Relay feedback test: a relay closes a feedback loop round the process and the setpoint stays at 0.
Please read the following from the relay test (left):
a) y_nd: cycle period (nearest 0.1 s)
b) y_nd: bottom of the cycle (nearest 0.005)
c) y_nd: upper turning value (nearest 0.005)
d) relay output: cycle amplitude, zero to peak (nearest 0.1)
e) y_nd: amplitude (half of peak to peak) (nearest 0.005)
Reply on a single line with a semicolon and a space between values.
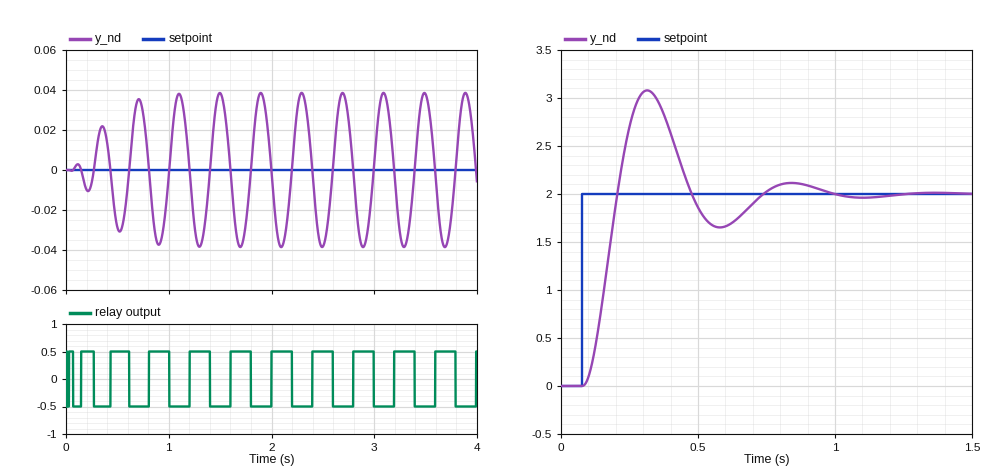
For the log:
0.4 s; -0.040; 0.040; 0.5; 0.040
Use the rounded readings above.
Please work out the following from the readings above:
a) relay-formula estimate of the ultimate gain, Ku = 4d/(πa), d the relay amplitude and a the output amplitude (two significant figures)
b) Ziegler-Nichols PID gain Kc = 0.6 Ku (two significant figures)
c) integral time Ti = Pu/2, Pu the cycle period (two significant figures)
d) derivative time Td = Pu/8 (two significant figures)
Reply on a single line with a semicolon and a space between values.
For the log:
16; 9.6; 0.20 s; 0.050 s
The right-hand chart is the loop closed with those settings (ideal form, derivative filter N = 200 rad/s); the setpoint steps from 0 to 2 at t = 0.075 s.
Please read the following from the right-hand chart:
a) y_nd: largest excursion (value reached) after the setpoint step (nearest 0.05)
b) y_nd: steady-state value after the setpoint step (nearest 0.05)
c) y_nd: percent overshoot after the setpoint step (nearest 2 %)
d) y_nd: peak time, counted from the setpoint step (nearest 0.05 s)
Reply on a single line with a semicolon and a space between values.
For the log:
3.10; 2.00; 54 %; 0.25 s
